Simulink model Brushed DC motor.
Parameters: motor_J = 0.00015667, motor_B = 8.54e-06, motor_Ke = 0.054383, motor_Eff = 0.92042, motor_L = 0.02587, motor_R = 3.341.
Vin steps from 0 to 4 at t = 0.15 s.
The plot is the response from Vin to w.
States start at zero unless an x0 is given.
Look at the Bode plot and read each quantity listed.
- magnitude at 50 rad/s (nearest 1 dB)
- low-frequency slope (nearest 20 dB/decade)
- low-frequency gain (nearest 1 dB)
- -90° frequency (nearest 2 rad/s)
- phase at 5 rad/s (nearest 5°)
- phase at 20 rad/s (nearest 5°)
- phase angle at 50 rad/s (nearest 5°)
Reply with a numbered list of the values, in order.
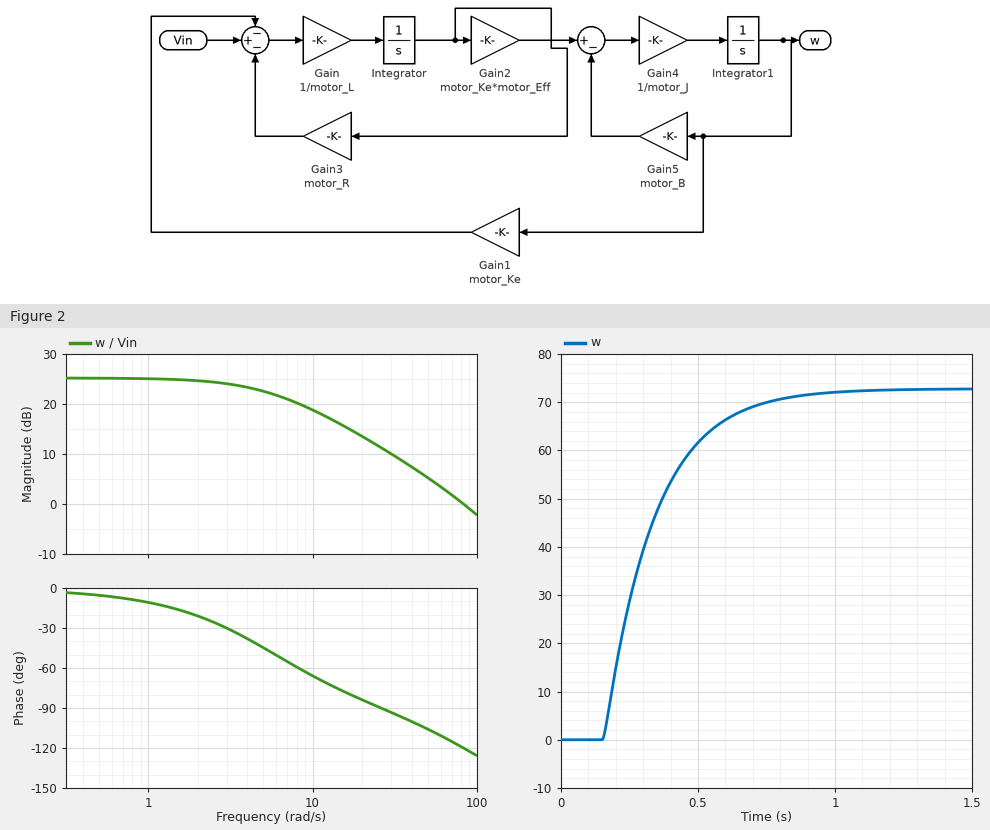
1. 5 dB
2. 0 dB/decade
3. 25 dB
4. 26 rad/s
5. -45°
6. -85°
7. -105°
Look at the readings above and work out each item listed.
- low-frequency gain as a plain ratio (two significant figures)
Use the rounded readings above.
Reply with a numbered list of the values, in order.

1. 18
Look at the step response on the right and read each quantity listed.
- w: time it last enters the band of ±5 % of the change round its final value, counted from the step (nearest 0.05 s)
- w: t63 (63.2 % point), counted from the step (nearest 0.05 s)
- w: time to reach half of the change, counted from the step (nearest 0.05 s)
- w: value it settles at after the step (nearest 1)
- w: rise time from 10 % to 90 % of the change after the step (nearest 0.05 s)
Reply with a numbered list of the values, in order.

1. 0.55 s
2. 0.20 s
3. 0.15 s
4. 73
5. 0.40 s
